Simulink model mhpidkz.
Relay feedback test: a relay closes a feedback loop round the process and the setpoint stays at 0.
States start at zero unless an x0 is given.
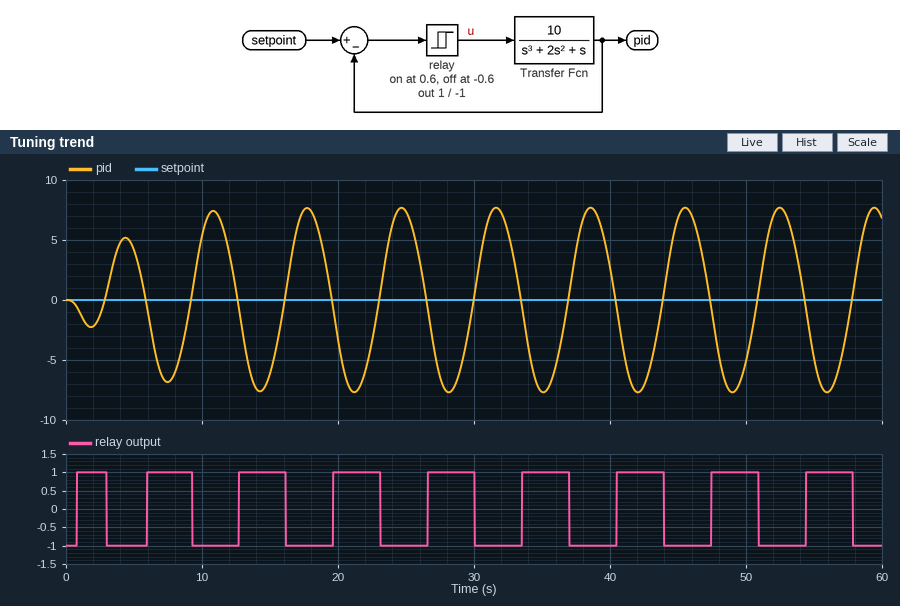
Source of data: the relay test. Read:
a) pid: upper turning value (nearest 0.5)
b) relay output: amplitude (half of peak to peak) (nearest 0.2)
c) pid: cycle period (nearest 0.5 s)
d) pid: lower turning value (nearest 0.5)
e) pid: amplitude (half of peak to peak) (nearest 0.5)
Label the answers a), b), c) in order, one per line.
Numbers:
a) 7.5
b) 1.0
c) 7.0 s
d) -7.5
e) 7.5
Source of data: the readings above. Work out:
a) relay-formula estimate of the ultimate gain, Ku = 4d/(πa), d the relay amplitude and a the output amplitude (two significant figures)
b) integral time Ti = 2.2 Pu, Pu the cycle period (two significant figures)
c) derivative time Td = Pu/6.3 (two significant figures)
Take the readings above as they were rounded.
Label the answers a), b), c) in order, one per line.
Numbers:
a) 0.17
b) 15 s
c) 1.1 s
